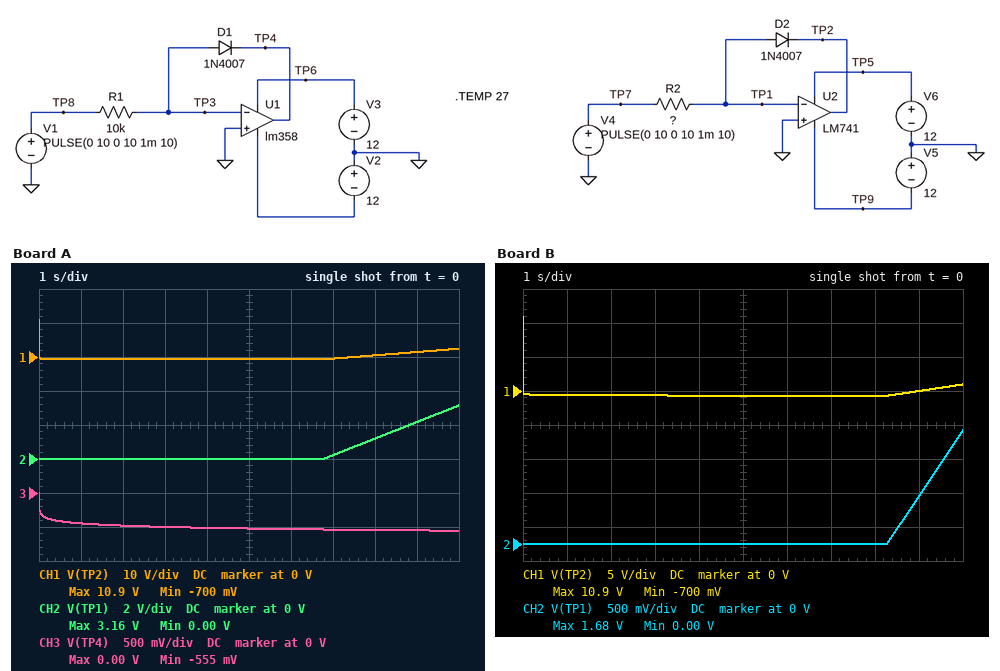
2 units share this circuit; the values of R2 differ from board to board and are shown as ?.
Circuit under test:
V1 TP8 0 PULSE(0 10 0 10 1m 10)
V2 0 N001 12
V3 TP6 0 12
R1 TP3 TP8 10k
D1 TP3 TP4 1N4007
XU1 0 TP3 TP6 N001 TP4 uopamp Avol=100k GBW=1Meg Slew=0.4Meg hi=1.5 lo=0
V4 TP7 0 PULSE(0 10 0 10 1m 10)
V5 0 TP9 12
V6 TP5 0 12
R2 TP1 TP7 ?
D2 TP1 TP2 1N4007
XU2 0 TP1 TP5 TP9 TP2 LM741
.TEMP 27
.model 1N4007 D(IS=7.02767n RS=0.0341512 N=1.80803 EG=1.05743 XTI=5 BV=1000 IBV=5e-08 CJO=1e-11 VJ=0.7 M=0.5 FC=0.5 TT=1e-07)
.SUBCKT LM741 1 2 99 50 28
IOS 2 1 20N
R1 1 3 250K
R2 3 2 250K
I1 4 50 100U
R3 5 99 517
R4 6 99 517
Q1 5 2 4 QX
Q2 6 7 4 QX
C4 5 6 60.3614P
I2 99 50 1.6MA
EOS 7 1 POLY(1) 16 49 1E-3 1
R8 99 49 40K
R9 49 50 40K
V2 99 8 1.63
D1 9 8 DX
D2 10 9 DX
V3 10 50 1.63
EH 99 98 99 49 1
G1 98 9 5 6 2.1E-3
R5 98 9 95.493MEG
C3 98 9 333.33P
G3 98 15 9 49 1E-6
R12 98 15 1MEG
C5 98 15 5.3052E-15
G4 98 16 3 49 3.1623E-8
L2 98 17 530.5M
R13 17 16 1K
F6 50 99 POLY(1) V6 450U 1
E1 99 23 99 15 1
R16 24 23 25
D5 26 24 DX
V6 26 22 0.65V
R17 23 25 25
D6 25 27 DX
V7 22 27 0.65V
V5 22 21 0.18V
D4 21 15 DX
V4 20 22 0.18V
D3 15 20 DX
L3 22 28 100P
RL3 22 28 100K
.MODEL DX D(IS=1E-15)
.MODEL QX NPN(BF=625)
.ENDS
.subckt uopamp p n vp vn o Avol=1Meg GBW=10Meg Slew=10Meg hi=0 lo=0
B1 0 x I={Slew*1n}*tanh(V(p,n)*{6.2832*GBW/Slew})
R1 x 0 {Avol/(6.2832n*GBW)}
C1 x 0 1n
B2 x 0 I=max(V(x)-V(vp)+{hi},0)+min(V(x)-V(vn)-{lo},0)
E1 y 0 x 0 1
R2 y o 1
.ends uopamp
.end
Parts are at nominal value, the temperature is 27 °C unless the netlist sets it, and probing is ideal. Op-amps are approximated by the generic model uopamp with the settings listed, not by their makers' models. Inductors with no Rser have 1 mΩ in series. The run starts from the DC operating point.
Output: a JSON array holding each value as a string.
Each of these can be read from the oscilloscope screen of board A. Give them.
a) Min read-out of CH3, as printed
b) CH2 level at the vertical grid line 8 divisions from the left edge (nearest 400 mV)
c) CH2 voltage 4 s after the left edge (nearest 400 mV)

["-555 mV", "1.2 V", "0 V"]
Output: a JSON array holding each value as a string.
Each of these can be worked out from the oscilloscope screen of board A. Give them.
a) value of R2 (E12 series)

["270 Ω"]
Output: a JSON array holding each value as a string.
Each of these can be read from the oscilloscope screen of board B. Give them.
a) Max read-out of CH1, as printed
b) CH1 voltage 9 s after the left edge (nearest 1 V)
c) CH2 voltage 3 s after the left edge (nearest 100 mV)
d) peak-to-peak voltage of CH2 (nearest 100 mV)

["10.9 V", "0 V", "0 V", "1.7 V"]
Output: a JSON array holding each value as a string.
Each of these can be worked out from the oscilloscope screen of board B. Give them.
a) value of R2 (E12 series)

["330 Ω"]
